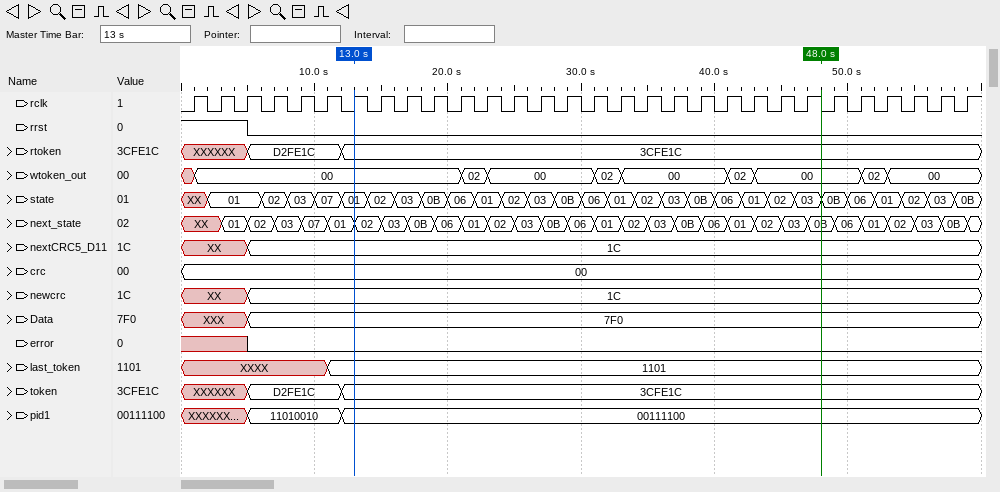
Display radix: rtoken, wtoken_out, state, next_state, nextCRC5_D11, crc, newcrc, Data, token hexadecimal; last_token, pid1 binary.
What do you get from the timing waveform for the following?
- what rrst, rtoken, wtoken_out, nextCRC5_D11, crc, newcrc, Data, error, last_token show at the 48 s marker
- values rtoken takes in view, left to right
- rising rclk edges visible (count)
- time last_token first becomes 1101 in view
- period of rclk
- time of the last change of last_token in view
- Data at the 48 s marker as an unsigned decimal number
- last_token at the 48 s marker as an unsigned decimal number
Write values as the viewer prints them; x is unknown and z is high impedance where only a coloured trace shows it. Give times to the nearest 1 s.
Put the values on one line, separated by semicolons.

rrst=0, rtoken=3CFE1C, wtoken_out=00, nextCRC5_D11=1C, crc=00, newcrc=1C, Data=7F0, error=0, last_token=1101; XXXXXX, D2FE1C, 3CFE1C; 30; 11 s; 2 s; 11 s; 2032; 13
